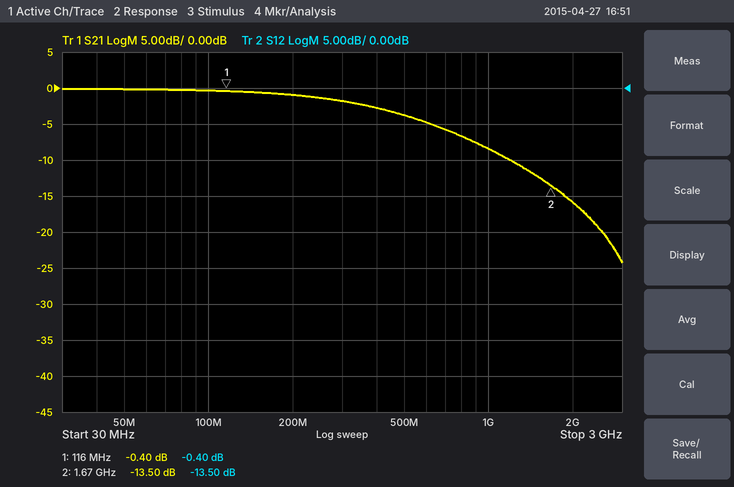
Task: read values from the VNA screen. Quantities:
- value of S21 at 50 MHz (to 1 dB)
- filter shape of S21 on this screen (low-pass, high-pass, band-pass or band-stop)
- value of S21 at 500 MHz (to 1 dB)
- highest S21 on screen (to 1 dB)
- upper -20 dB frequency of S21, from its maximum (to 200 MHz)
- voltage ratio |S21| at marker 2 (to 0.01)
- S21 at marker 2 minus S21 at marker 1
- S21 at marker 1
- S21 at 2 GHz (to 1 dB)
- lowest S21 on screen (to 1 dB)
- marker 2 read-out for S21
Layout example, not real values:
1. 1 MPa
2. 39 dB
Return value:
1. 0 dB
2. low-pass
3. -4 dB
4. 0 dB
5. 2.6 GHz
6. 0.21
7. -13.10 dB
8. -0.40 dB
9. -16 dB
10. -24 dB
11. -13.50 dB
